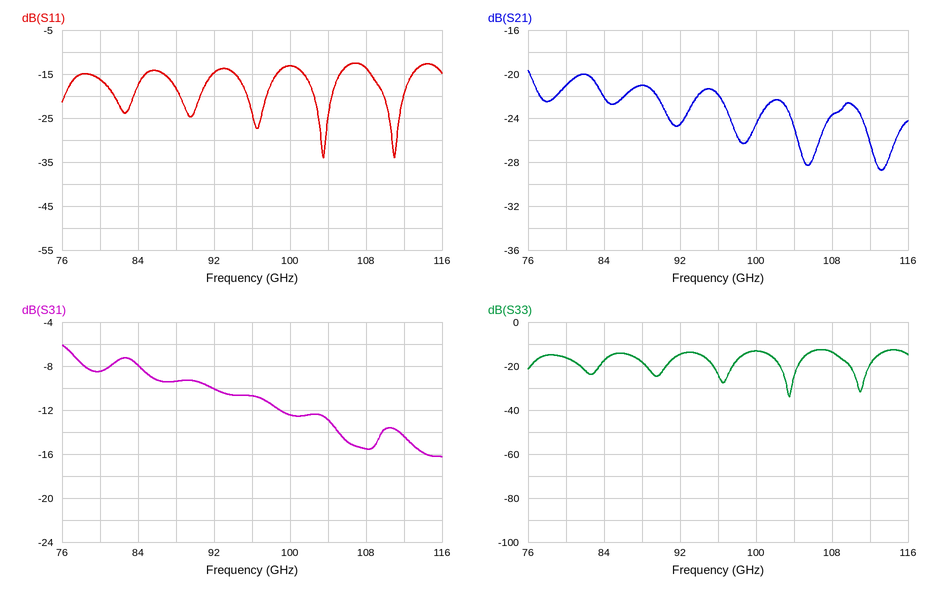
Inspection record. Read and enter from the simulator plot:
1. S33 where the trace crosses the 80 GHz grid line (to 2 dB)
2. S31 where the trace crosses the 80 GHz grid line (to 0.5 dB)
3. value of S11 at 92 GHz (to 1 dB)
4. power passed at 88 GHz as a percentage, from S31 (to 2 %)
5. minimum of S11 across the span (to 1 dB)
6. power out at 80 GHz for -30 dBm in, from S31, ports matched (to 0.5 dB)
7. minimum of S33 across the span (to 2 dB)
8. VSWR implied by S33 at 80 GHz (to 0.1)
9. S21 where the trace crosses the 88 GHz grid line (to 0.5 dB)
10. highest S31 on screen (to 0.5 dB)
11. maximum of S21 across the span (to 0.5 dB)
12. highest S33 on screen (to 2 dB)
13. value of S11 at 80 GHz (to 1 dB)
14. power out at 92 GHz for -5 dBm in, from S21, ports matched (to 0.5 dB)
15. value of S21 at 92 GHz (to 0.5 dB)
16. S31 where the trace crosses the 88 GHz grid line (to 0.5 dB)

-16 dB
-8.5 dB
-15 dB
12 %
-34 dB
-38.5 dBm
-34 dB
1.4
-21.0 dB
-6.0 dB
-19.5 dB
-12 dB
-16 dB
-29.5 dBm
-24.5 dB
-9.5 dB
